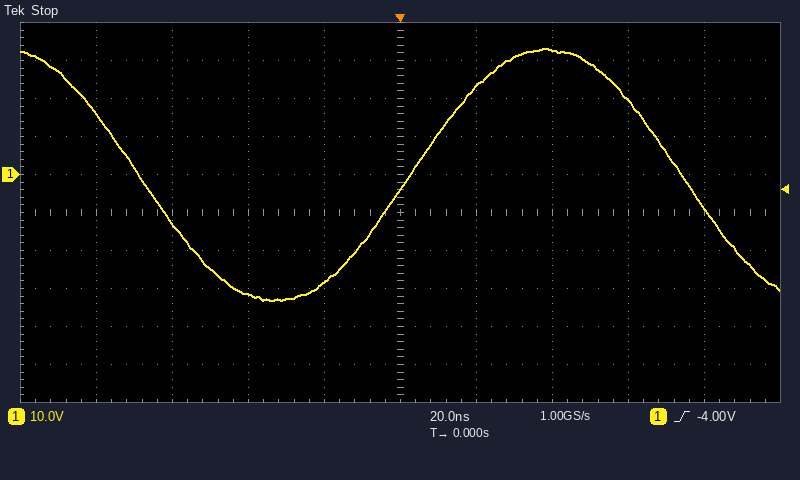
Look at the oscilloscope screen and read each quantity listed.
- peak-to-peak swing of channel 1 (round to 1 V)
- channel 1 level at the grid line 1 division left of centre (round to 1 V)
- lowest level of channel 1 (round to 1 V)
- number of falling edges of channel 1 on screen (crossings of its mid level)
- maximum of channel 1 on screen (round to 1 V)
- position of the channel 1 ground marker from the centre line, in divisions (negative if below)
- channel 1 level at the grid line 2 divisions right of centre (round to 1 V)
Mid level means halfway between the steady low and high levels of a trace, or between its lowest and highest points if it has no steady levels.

66 V
-28 V
-33 V
2
33 V
+1.0 div
33 V
